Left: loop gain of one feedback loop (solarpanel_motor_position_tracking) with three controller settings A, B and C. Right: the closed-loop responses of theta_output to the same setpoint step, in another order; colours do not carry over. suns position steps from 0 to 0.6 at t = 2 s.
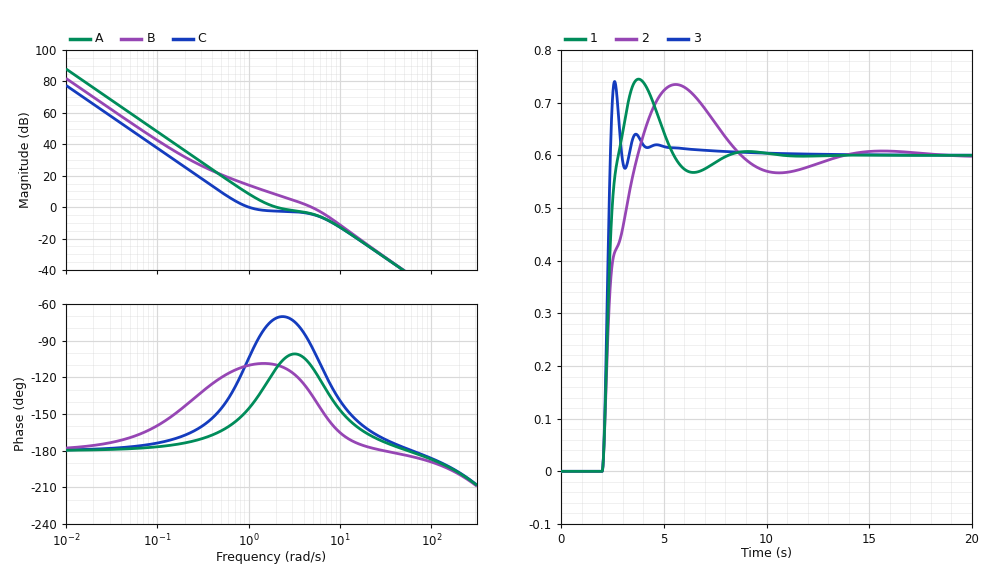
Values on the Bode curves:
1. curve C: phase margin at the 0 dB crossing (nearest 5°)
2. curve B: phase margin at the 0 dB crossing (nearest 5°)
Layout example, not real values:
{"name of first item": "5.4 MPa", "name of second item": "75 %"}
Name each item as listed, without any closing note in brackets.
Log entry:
{"curve C: phase margin at the 0 dB crossing": "75°", "curve B: phase margin at the 0 dB crossing": "45°"}
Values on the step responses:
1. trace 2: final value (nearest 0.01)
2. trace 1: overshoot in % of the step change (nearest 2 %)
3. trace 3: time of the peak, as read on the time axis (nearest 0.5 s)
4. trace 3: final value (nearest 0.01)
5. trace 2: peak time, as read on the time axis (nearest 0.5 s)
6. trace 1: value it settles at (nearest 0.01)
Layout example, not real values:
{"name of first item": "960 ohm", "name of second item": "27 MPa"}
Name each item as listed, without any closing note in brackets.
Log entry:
{"trace 2: final value": "0.60", "trace 1: overshoot in % of the step change": "24 %", "trace 3: time of the peak, as read on the time axis": "2.5 s", "trace 3: final value": "0.60", "trace 2: peak time, as read on the time axis": "5.5 s", "trace 1: value it settles at": "0.60"}
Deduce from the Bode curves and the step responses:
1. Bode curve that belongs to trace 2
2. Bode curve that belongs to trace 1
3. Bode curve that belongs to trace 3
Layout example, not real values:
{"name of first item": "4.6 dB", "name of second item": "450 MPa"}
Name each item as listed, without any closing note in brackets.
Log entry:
{"Bode curve that belongs to trace 2": "C", "Bode curve that belongs to trace 1": "A", "Bode curve that belongs to trace 3": "B"}
